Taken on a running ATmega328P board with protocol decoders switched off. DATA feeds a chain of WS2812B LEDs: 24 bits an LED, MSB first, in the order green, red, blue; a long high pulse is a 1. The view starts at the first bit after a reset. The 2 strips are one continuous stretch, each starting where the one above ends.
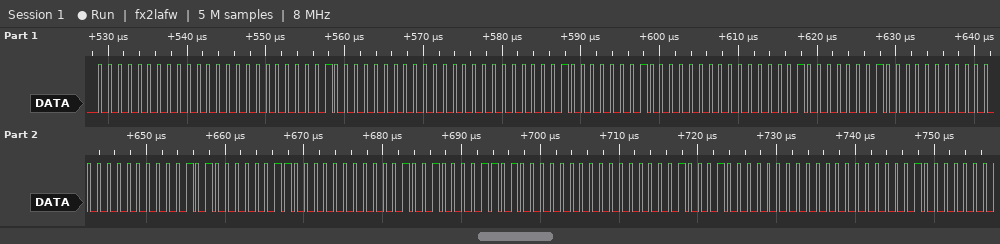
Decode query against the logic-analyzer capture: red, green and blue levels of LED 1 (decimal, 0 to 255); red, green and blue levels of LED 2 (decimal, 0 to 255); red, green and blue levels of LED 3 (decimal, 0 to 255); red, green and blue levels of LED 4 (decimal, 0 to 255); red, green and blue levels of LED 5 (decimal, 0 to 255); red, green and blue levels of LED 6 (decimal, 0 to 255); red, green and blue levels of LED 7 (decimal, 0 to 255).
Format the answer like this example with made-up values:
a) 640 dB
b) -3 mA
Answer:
a) 0, 0, 1
b) 0, 0, 1
c) 0, 1, 1
d) 0, 1, 0
e) 3, 5, 0
f) 26, 18, 0
g) 16, 1, 0
